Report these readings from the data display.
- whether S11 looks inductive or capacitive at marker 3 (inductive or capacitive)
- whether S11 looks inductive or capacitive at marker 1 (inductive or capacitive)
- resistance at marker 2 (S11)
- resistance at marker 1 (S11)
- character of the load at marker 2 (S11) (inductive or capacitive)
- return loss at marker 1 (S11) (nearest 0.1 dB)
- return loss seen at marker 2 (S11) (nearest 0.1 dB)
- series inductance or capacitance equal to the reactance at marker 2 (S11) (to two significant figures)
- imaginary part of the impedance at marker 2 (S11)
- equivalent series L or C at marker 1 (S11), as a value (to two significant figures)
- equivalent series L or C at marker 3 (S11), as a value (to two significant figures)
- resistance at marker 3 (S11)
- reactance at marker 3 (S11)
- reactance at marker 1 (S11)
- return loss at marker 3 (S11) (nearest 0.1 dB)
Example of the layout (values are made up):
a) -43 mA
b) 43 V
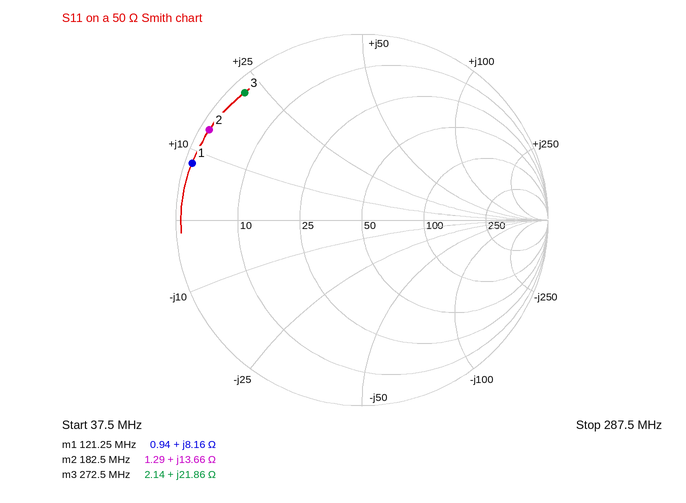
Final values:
a) inductive
b) inductive
c) 1.29 Ω
d) 0.94 Ω
e) inductive
f) 0.3 dB
g) 0.4 dB
h) 12 nH
i) +13.66 Ω
j) 11 nH
k) 13 nH
l) 2.14 Ω
m) +21.86 Ω
n) +8.16 Ω
o) 0.6 dB
